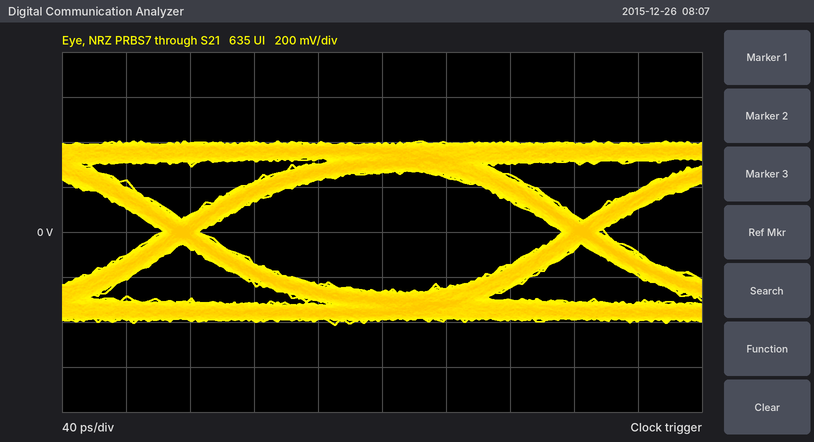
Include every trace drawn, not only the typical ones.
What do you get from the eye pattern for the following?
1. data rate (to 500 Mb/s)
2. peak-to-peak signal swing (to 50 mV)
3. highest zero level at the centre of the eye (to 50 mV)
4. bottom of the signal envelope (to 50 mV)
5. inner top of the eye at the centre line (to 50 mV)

4.0 Gb/s
800 mV
-250 mV
-400 mV
250 mV
